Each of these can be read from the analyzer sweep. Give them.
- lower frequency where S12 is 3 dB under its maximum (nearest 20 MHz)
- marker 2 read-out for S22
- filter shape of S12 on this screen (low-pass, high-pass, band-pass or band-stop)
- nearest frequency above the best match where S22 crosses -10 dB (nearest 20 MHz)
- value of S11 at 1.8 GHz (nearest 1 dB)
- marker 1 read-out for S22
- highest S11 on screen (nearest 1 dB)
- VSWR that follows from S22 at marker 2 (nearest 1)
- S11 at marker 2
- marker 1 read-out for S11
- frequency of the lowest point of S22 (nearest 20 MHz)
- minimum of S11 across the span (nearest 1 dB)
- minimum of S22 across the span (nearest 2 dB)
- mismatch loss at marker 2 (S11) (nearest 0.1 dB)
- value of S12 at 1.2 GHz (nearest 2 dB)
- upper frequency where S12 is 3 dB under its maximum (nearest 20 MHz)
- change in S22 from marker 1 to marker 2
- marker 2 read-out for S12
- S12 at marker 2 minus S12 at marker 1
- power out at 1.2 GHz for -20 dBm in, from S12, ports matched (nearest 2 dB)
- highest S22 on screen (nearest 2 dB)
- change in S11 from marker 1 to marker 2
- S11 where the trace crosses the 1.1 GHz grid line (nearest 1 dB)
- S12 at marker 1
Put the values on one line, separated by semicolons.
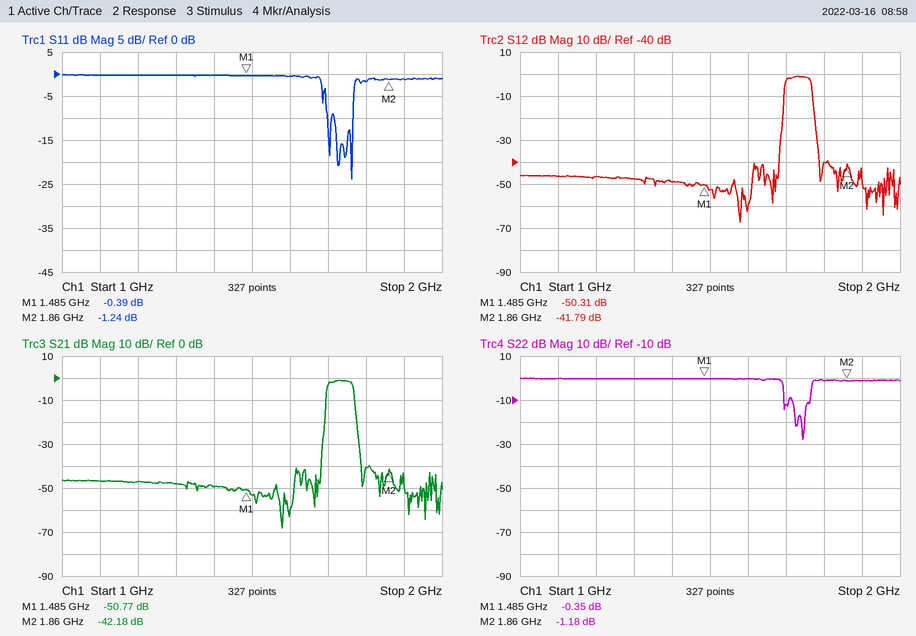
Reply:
1.70 GHz; -1.18 dB; band-pass; 1.76 GHz; -2 dB; -0.35 dB; 0 dB; 15; -1.24 dB; -0.39 dB; 1.74 GHz; -24 dB; -28 dB; 6.0 dB; -46 dB; 1.76 GHz; -0.83 dB; -41.79 dB; 8.52 dB; -66 dBm; 0 dB; -0.85 dB; 0 dB; -50.31 dB
